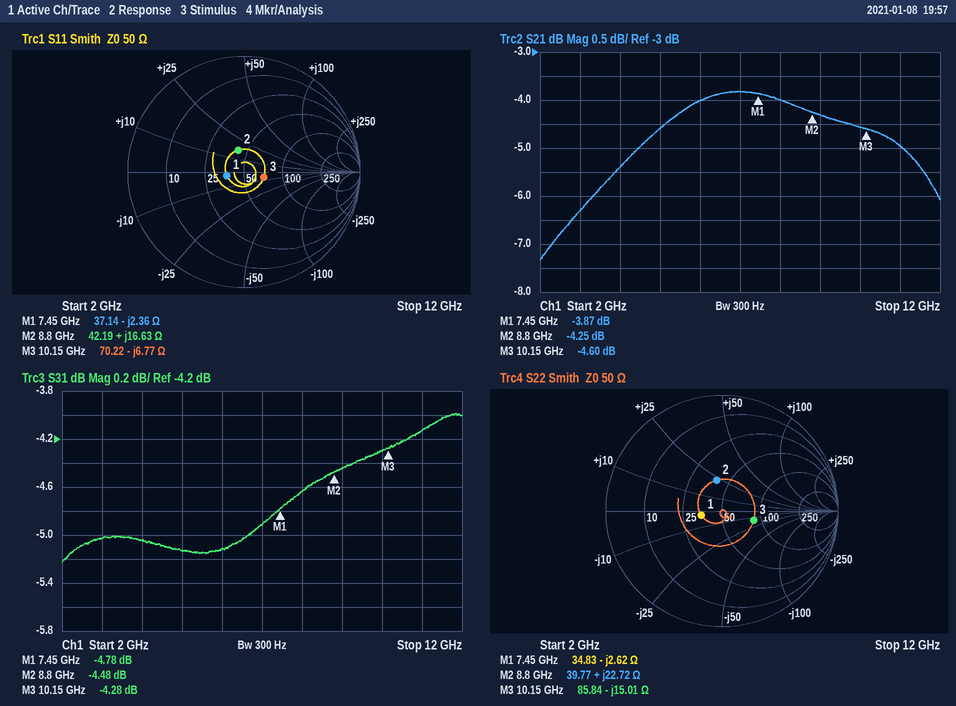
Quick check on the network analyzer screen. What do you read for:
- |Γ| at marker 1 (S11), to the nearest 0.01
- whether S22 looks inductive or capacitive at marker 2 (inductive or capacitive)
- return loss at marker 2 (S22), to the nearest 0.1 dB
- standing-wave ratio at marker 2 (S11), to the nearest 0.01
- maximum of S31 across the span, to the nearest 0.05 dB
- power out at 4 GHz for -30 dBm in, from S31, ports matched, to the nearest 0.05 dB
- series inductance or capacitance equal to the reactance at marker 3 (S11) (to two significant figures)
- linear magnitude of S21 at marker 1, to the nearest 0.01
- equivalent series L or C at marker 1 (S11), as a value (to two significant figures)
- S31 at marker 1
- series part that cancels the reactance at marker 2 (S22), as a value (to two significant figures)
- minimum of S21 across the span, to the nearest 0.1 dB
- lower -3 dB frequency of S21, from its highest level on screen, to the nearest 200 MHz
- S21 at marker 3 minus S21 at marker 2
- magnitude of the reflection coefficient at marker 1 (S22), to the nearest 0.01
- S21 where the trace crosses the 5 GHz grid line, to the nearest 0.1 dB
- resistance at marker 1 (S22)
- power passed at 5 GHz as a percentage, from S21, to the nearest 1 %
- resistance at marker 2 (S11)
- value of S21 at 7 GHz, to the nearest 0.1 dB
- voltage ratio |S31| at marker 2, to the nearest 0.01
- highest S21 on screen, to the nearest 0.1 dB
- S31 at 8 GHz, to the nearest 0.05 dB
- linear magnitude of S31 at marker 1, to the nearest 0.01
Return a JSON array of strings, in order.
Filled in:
["0.15", "inductive", "11.4 dB", "1.49", "-4.00 dB", "-35.05 dBm", "2.3 pF", "0.64", "9.1 pF", "-4.78 dB", "800 fF", "-7.3 dB", "2.4 GHz", "-0.35 dB", "0.18", "-4.6 dB", "34.83 Ω", "35 %", "42.19 Ω", "-3.8 dB", "0.60", "-3.8 dB", "-4.65 dB", "0.58"]
